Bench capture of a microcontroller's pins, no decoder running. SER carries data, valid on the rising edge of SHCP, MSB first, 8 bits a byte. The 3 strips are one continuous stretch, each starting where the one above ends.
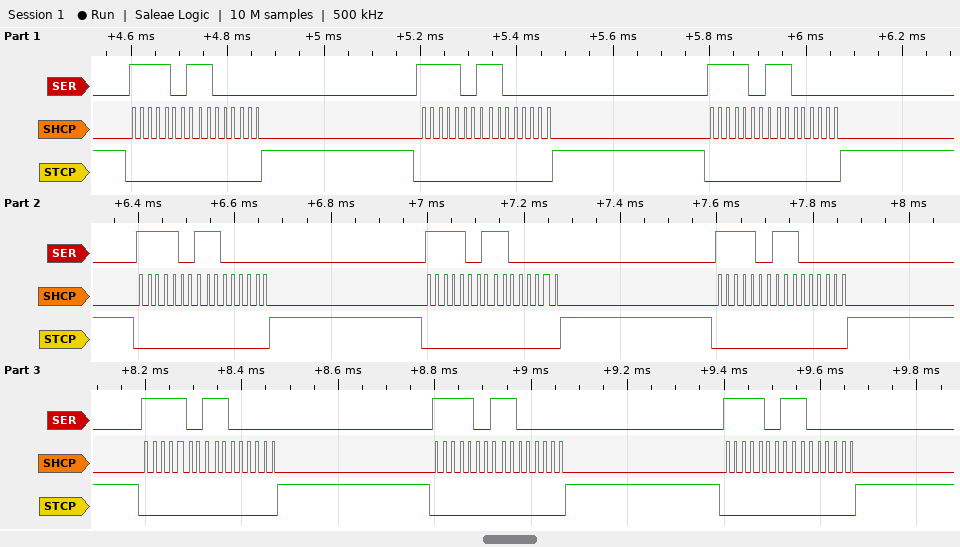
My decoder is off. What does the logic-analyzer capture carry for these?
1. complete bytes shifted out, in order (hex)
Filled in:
0xF9 0xC0 0xF9 0xC0 0xF9 0xC0 0xF9 0xC0 0xF9 0xC0 0xF9 0xC0 0xF9 0xC0 0xF9 0xC0 0xF9 0xC0
